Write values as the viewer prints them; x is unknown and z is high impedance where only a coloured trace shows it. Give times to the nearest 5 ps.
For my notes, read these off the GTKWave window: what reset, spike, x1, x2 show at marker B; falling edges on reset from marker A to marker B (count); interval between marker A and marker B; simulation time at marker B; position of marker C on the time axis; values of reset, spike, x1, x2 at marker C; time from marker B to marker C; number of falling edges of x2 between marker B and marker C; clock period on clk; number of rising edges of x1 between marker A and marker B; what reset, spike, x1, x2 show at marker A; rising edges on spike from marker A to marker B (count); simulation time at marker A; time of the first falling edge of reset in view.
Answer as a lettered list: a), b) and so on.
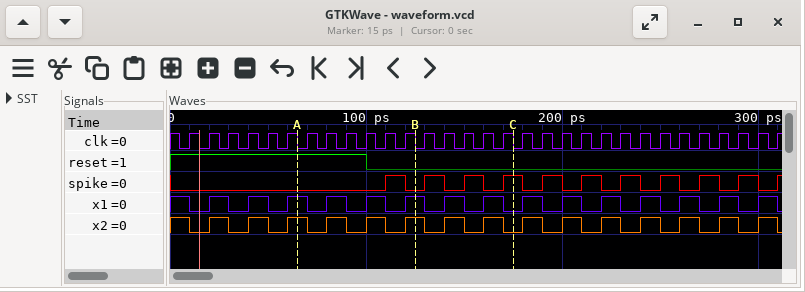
a) reset=0, spike=0, x1=1, x2=1
b) 1
c) 60 ps
d) 125 ps
e) 175 ps
f) reset=0, spike=1, x1=0, x2=0
g) 50 ps
h) 3
i) 10 ps
j) 3
k) reset=1, spike=0, x1=1, x2=1
l) 1
m) 65 ps
n) 100 ps
